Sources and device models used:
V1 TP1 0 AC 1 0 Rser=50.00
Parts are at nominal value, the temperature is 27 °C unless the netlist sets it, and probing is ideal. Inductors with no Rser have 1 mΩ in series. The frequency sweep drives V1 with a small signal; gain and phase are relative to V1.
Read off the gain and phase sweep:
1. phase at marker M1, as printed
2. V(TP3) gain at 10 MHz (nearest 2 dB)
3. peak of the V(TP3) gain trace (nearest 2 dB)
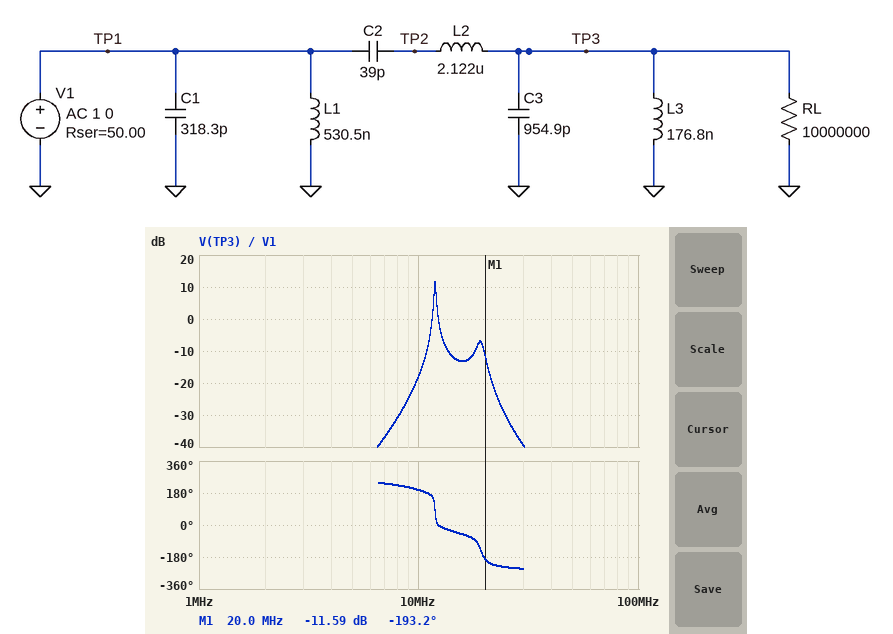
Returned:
-193.2 deg
-18 dB
12 dB
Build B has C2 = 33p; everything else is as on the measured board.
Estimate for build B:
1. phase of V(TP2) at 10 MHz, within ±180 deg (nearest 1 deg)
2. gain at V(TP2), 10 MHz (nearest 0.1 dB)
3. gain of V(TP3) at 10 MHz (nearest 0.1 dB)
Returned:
-161 deg
-6.0 dB
-20.0 dB
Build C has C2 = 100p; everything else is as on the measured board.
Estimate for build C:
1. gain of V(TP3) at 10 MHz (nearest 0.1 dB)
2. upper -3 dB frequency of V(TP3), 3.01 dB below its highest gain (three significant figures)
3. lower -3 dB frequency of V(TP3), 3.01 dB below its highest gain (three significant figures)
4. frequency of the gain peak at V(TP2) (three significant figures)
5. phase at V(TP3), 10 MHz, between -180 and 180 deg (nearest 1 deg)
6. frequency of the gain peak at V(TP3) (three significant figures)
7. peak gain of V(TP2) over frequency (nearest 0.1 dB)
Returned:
-4.2 dB
14.1 MHz
12.2 MHz
9.31 MHz
82 deg
13.3 MHz
11.1 dB
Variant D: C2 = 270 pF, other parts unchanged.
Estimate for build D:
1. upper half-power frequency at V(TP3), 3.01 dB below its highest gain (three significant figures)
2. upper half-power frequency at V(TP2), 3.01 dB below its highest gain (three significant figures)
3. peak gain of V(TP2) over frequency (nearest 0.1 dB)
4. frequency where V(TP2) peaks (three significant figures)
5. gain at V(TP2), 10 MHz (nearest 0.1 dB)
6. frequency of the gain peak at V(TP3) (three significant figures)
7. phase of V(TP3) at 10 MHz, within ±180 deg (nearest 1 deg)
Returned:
13.1 MHz
5.98 MHz
11.7 dB
5.69 MHz
0.9 dB
12.9 MHz
44 deg
